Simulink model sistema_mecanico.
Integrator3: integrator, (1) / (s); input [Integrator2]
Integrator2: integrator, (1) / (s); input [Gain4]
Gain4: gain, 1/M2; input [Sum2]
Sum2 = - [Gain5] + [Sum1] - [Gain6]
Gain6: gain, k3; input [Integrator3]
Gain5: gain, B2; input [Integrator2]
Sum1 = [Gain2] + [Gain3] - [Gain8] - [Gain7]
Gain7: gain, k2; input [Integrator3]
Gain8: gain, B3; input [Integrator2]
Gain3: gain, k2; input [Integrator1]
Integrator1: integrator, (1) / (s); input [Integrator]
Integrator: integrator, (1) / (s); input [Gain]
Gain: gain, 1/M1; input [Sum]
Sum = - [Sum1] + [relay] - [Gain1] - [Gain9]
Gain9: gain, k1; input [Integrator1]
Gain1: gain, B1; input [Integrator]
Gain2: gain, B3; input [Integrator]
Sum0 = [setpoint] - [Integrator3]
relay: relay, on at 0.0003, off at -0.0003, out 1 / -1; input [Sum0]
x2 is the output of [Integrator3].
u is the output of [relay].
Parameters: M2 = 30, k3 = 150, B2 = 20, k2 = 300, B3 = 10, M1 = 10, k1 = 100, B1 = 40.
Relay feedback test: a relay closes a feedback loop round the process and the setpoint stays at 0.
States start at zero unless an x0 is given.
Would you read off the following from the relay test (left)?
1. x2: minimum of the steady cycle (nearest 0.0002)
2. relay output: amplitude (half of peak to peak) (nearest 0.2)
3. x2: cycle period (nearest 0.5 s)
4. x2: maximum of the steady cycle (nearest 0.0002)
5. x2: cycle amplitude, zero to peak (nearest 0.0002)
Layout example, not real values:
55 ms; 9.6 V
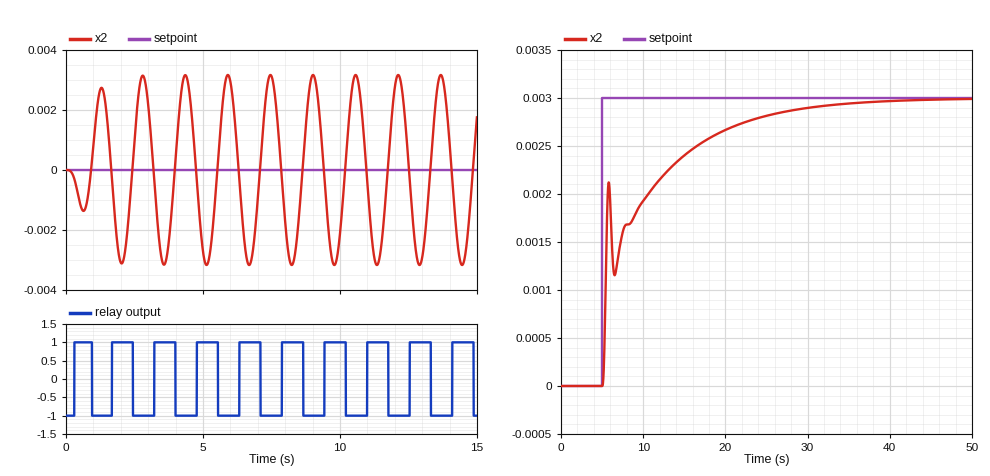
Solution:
-0.0032; 1.0; 1.5 s; 0.0032; 0.0032
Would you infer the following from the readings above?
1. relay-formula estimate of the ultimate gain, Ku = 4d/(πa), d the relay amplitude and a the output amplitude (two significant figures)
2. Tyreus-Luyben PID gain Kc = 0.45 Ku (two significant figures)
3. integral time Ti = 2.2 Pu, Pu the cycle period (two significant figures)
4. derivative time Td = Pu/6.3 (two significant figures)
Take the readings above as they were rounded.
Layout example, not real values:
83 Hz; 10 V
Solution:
400; 180; 3.3 s; 0.24 s
